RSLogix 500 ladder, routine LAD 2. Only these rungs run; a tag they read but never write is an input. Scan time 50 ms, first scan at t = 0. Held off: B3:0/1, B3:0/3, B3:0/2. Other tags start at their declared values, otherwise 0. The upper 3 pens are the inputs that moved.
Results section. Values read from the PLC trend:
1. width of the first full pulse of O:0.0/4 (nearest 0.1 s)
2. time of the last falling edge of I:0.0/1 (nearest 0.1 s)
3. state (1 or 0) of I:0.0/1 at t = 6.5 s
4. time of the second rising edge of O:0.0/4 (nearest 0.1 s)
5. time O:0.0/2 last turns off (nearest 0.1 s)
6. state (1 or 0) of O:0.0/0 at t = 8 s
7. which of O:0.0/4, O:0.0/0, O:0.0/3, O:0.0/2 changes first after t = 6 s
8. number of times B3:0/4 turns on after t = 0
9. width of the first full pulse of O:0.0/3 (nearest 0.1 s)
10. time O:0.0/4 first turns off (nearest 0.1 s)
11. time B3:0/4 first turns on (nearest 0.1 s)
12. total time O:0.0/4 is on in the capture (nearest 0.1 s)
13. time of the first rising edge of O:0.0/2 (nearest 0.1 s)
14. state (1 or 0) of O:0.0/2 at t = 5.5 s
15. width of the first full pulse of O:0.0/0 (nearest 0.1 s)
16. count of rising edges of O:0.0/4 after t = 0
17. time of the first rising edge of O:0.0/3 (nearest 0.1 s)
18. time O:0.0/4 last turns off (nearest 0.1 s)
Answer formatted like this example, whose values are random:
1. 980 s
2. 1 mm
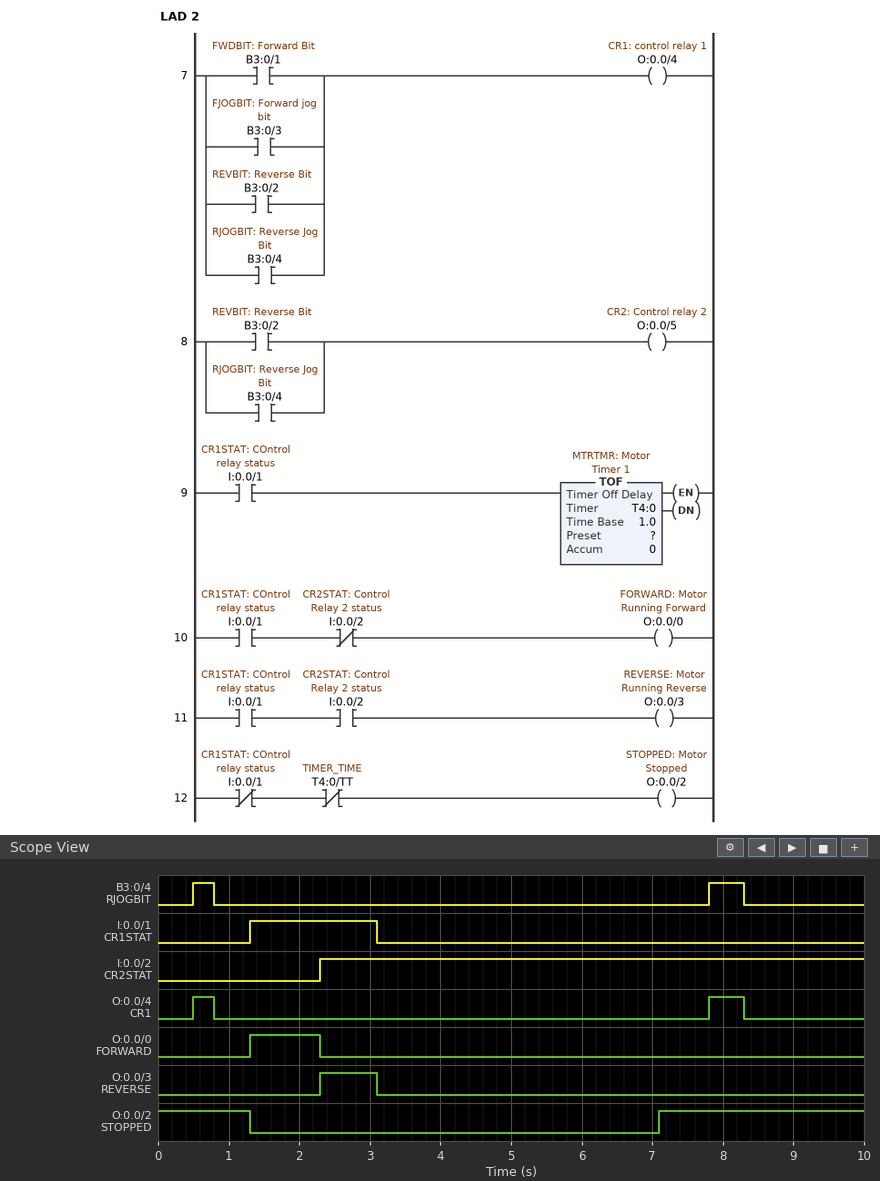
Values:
1. 0.3 s
2. 3.1 s
3. 0
4. 7.8 s
5. 1.3 s
6. 0
7. O:0.0/2
8. 2
9. 0.8 s
10. 0.8 s
11. 0.5 s
12. 0.8 s
13. 7.1 s
14. 0
15. 1.0 s
16. 2
17. 2.3 s
18. 8.3 s
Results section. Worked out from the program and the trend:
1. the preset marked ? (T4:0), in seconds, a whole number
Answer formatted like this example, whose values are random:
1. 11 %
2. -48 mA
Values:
1. 4 s
